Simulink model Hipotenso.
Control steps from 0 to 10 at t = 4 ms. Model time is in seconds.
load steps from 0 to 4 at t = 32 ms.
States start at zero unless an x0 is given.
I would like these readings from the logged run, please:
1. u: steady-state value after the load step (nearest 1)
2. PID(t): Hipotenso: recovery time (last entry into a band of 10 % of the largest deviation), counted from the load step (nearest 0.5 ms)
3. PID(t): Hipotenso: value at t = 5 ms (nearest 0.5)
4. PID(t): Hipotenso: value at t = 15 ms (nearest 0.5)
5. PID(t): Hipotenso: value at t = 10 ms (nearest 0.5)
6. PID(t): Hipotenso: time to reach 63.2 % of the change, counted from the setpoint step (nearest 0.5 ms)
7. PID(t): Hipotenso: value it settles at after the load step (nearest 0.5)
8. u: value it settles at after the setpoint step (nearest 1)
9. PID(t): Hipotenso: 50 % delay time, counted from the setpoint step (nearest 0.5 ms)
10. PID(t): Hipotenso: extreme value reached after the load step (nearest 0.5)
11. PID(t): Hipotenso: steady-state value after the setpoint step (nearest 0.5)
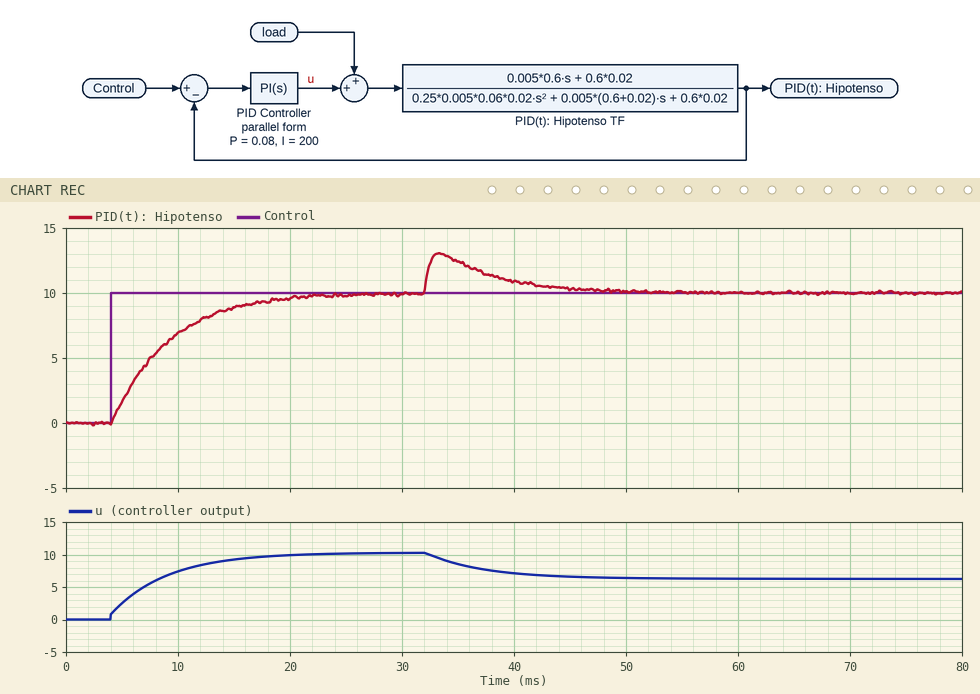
6
13.5 ms
1.5
9.0
7.0
5.0 ms
10.0
10
3.5 ms
13.0
10.0
